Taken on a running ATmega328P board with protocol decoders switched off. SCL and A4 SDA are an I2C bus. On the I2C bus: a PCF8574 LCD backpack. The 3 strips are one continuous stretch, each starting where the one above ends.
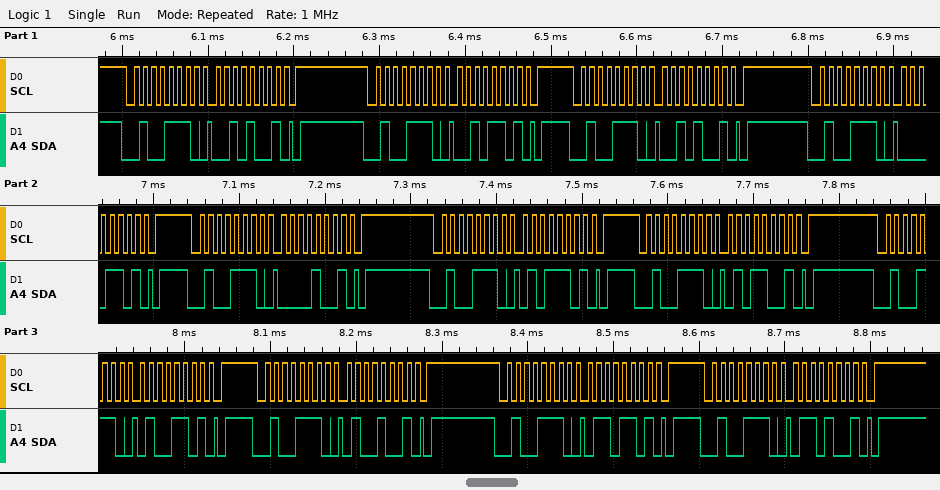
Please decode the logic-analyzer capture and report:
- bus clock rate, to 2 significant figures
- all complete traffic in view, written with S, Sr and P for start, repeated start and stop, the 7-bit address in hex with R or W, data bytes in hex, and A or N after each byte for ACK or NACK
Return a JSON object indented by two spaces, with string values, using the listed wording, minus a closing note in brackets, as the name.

{
  "bus clock rate, to 2 significant figures": "100 kHz",
  "all complete traffic in view, written with S, Sr and P for start, repeated start and stop, the 7-bit address in hex with R or W, data bytes in hex, and A or N after each byte for ACK or NACK": "S 27W A 29 A P S 27W A 2D A P S 27W A 29 A P S 27W A 0D A P S 27W A 09 A P S 27W A 5D A P S 27W A 59 A P S 27W A 4D A P S 27W A 49 A P S 27W A 6D A P S 27W A 69 A P"
}
